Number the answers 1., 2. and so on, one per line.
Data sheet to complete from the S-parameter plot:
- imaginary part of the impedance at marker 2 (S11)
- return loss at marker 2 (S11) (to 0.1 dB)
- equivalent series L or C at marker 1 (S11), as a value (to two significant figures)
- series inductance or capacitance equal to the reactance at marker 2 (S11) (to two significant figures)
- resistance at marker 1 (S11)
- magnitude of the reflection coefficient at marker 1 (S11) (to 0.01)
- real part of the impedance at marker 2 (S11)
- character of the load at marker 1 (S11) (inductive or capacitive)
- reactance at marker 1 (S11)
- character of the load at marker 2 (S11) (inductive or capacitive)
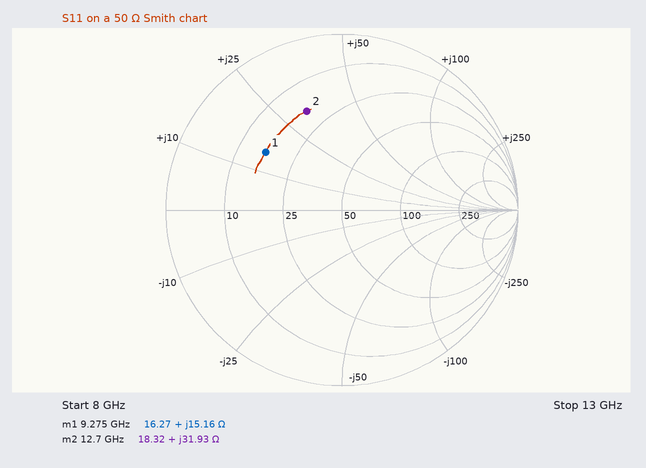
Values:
1. +31.93 Ω
2. 4.5 dB
3. 260 pH
4. 400 pH
5. 16.27 Ω
6. 0.54
7. 18.32 Ω
8. inductive
9. +15.16 Ω
10. inductive
